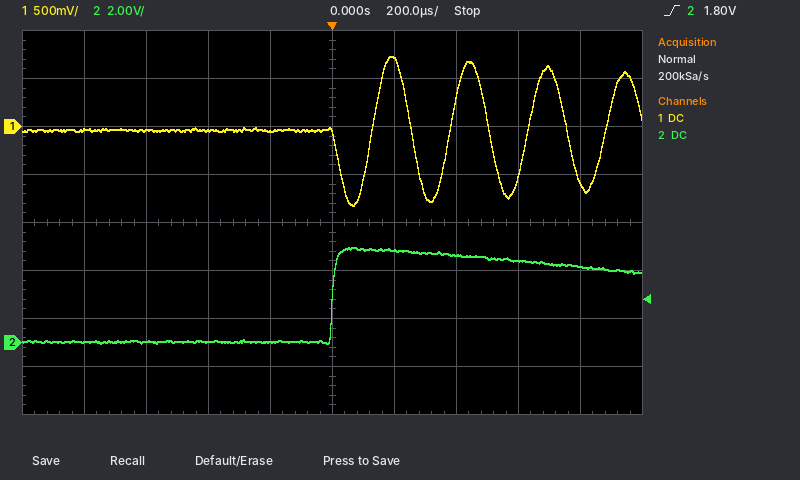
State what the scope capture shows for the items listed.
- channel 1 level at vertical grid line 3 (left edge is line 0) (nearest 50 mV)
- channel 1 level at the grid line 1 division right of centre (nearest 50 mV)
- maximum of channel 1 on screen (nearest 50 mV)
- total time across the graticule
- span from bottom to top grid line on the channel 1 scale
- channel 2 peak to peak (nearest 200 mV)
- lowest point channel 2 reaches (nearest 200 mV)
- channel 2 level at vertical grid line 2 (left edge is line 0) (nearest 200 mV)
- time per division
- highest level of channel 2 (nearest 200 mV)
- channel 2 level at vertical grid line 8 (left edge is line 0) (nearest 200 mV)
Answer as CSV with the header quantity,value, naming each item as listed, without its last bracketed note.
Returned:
quantity,value
channel 1 level at vertical grid line 3 (left edge is line 0),-50 mV
channel 1 level at the grid line 1 division right of centre,700 mV
maximum of channel 1 on screen,750 mV
total time across the graticule,2 ms
span from bottom to top grid line on the channel 1 scale,4 V
channel 2 peak to peak,4.0 V
lowest point channel 2 reaches,0.0 V
channel 2 level at vertical grid line 2 (left edge is line 0),0.0 V
time per division,200 µs
highest level of channel 2,4.0 V
channel 2 level at vertical grid line 8 (left edge is line 0),3.4 V
